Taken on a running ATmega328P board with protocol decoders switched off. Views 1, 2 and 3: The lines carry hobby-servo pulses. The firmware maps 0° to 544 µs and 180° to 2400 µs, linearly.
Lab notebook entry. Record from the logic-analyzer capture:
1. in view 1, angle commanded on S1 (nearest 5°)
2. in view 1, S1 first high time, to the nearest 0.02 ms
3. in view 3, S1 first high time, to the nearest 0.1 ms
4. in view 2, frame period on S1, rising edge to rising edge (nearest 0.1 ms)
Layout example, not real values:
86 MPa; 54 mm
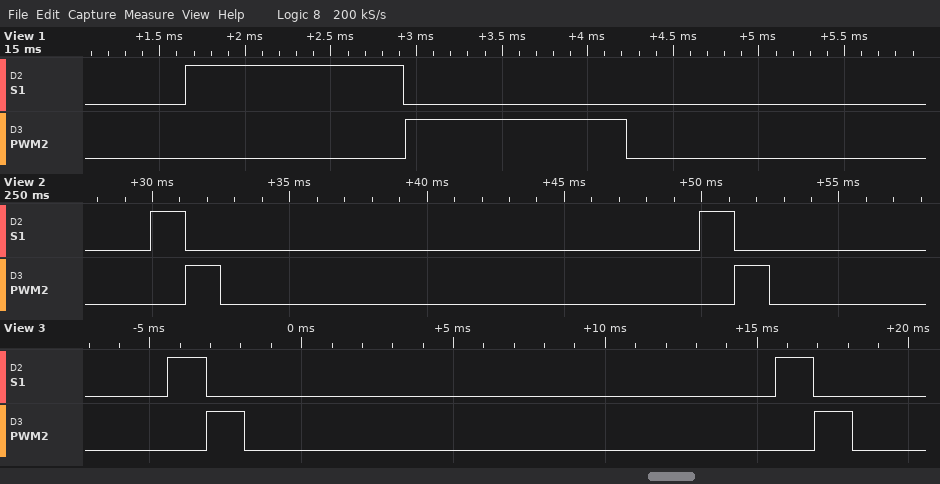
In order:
70°; 1.28 ms; 1.3 ms; 20.0 ms
